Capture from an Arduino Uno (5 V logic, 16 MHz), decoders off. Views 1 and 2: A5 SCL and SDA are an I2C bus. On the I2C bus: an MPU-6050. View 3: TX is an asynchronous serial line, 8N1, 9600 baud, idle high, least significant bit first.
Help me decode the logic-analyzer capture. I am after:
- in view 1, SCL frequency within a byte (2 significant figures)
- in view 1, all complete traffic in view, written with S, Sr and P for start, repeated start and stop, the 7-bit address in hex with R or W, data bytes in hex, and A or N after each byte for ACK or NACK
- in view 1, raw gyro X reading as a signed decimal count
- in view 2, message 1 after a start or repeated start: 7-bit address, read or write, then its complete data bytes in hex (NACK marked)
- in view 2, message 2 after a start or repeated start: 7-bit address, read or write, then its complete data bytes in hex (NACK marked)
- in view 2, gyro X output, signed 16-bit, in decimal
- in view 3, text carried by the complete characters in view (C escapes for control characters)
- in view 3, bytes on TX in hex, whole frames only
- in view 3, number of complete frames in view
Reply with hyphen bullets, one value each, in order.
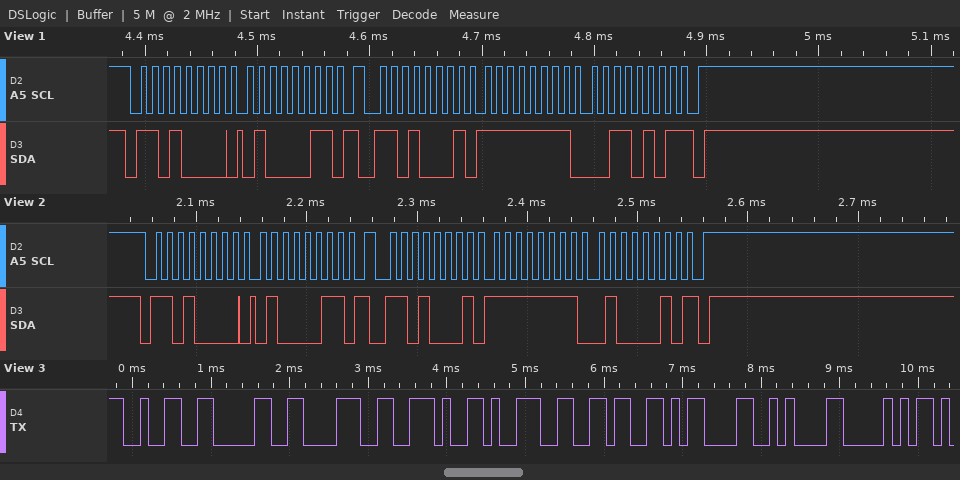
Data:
- 100 kHz
- S 68W A 43 A Sr 68R A FF A 35 N P
- -203
- 0x68 write: 43
- 0x68 read: FF 42 NACK
- -190
- "208.96\r\nP"
- 32 30 38 2E 39 36 0D 0A 50
- 9
